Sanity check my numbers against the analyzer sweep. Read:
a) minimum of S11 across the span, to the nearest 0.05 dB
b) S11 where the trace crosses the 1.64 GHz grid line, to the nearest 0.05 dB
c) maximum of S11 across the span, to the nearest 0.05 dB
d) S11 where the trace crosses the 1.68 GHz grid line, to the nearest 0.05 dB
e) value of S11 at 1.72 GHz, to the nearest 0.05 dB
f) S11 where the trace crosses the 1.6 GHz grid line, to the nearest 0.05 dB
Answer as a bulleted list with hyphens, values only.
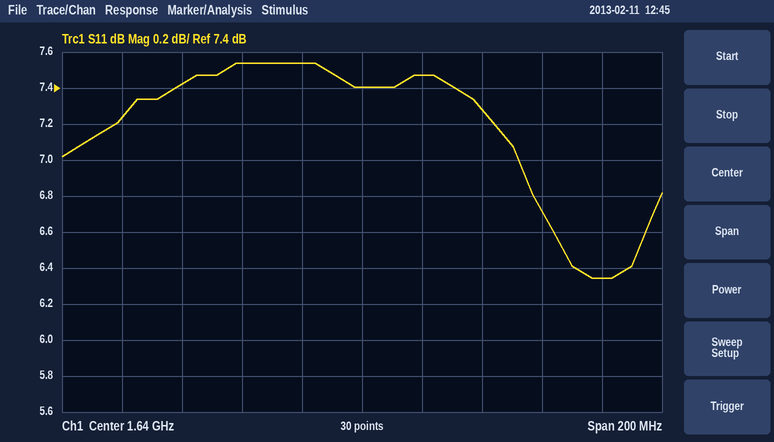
- 6.35 dB
- 7.40 dB
- 7.55 dB
- 7.30 dB
- 6.35 dB
- 7.55 dB
